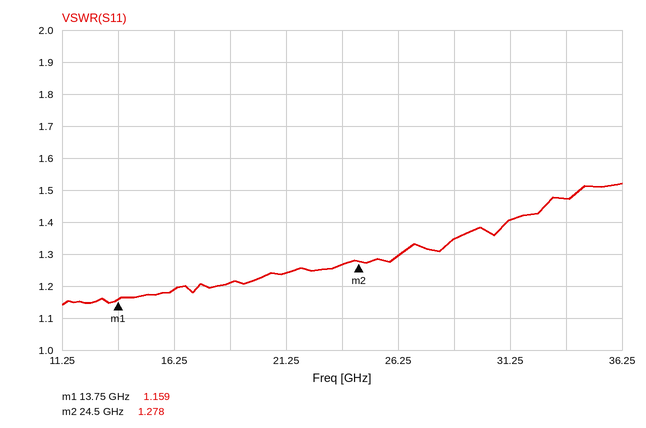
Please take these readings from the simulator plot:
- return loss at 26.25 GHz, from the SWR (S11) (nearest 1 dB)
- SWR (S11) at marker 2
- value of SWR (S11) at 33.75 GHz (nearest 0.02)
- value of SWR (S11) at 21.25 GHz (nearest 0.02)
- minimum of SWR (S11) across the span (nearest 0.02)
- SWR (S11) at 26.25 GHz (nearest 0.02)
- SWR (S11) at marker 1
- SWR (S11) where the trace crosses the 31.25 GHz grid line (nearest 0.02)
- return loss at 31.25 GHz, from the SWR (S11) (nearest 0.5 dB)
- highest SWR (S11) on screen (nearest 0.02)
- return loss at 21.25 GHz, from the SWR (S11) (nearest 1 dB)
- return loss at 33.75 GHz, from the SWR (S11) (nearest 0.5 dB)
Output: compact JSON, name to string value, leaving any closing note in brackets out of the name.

{"return loss at 26.25 GHz, from the SWR (S11)": "18 dB", "SWR (S11) at marker 2": "1.278", "value of SWR (S11) at 33.75 GHz": "1.48", "value of SWR (S11) at 21.25 GHz": "1.24", "minimum of SWR (S11) across the span": "1.14", "SWR (S11) at 26.25 GHz": "1.30", "SWR (S11) at marker 1": "1.159", "SWR (S11) where the trace crosses the 31.25 GHz grid line": "1.40", "return loss at 31.25 GHz, from the SWR (S11)": "15.5 dB", "highest SWR (S11) on screen": "1.52", "return loss at 21.25 GHz, from the SWR (S11)": "19 dB", "return loss at 33.75 GHz, from the SWR (S11)": "14.5 dB"}
